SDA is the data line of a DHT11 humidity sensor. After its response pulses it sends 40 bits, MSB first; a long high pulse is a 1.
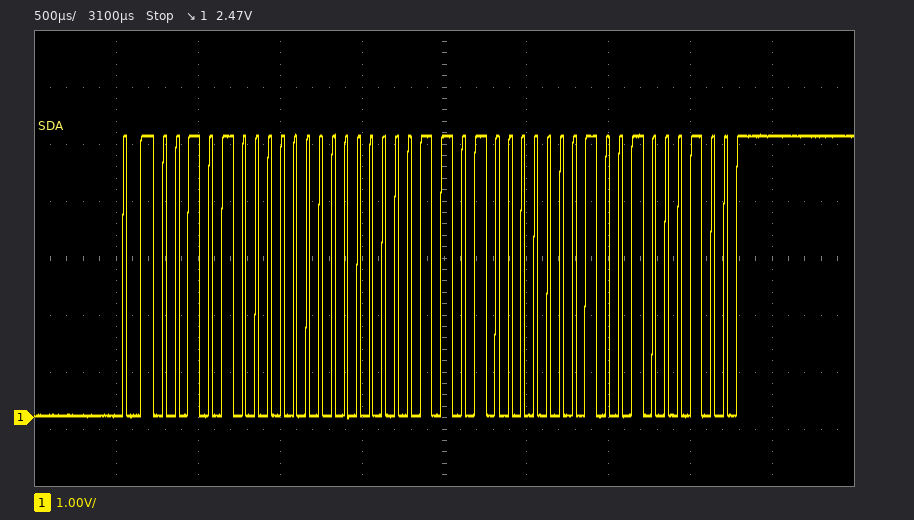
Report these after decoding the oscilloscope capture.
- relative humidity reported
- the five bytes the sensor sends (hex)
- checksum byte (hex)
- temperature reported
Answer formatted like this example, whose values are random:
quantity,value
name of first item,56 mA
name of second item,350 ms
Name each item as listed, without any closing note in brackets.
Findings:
quantity,value
relative humidity reported,40 %
the five bytes the sensor sends,28 00 1A 02 44
checksum byte,0x44
temperature reported,26.2 °C
